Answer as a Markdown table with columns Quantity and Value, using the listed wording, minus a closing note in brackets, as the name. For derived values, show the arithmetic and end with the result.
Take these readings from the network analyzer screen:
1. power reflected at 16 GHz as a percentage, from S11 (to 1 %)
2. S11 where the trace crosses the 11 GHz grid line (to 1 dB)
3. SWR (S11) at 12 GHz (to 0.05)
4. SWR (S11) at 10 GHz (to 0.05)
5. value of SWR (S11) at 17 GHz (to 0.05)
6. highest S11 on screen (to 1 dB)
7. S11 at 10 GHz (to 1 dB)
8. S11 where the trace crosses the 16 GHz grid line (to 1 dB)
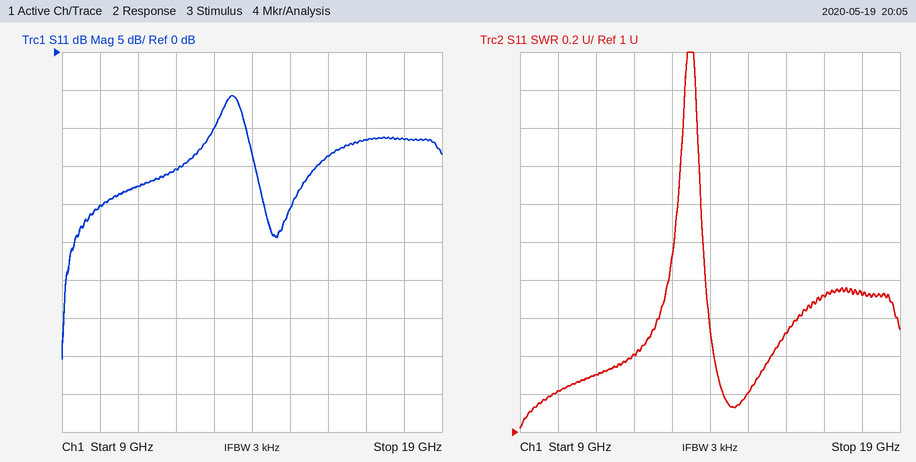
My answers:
| Quantity | Value |
|---|---|
| power reflected at 16 GHz as a percentage, from S11 | 10^(-14/10) ≈ 4 % |
| S11 where the trace crosses the 11 GHz grid line | -18 dB |
| SWR (S11) at 12 GHz | 1.40 |
| SWR (S11) at 10 GHz | 1.20 |
| value of SWR (S11) at 17 GHz | 1.70 |
| highest S11 on screen | -6 dB |
| S11 at 10 GHz | -20 dB |
| S11 where the trace crosses the 16 GHz grid line | -14 dB |
